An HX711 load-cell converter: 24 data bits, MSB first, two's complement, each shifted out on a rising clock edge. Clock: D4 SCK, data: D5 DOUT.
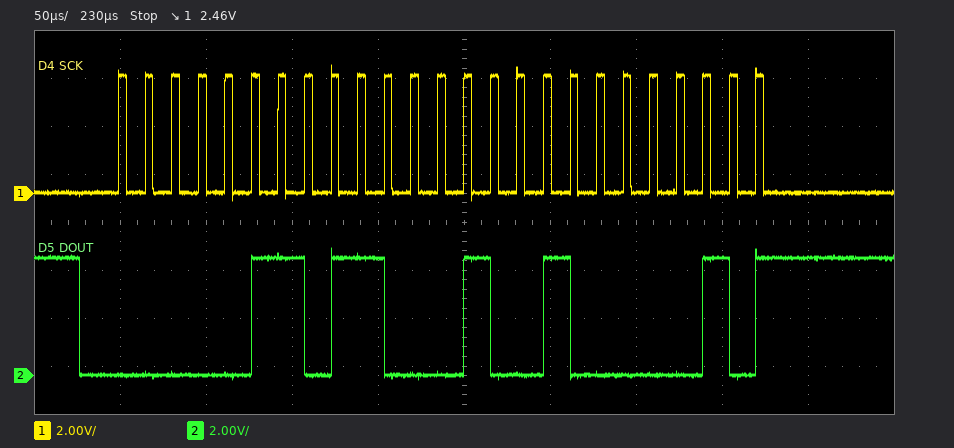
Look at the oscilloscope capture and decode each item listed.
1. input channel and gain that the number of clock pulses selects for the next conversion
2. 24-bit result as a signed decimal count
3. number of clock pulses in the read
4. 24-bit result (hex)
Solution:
channel A, gain 128
443522
25
0x06C482
